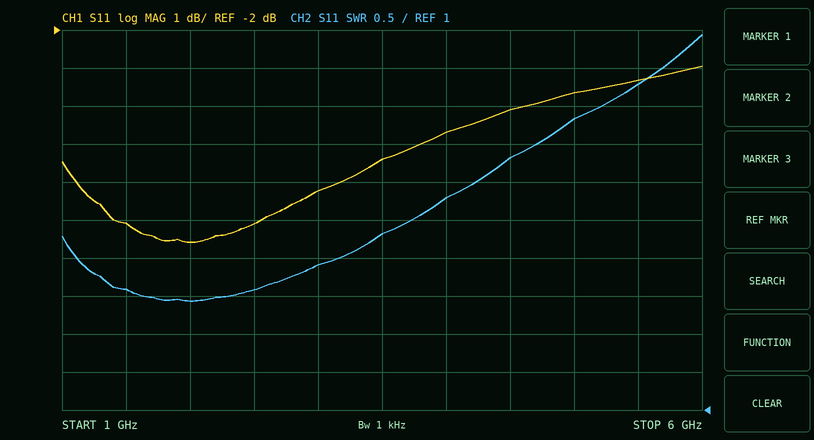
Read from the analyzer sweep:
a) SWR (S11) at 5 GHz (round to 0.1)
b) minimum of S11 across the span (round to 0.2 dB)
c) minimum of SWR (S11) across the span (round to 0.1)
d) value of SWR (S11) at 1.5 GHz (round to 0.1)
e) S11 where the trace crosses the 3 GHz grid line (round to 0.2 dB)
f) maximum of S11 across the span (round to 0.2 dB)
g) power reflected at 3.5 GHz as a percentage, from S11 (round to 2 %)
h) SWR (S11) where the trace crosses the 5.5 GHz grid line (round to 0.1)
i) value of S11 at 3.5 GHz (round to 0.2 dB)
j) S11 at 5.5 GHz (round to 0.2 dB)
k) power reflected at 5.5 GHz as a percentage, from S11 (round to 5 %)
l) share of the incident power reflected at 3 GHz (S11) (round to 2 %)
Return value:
4.8
-7.6 dB
2.4
2.6
-6.2 dB
-3.0 dB
28 %
5.3
-5.4 dB
-3.4 dB
45 %
24 %
